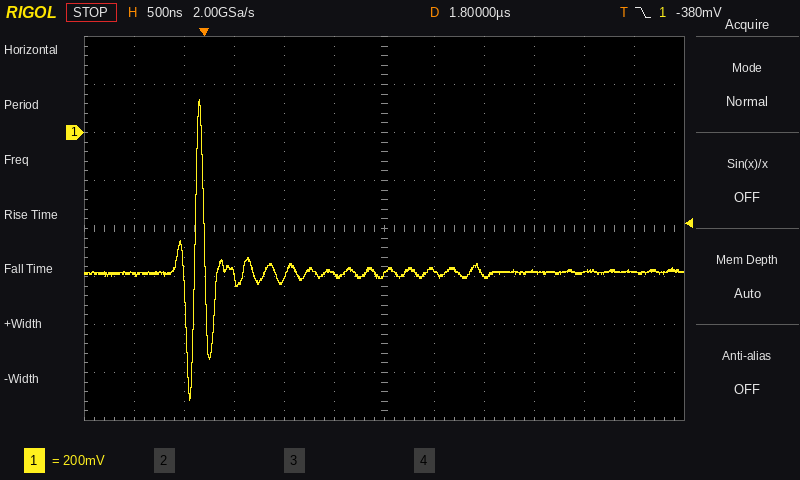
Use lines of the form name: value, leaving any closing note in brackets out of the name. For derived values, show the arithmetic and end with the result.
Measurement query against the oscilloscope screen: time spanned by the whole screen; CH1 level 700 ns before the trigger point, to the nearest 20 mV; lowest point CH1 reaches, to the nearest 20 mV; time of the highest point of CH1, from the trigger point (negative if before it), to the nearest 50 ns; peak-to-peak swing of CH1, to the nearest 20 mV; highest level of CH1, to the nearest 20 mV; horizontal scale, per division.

time spanned by the whole screen: 6 µs
CH1 level 700 ns before the trigger point, to the nearest 20 mV: -600 mV
lowest point CH1 reaches, to the nearest 20 mV: -1.12 V
time of the highest point of CH1, from the trigger point (negative if before it), to the nearest 50 ns: -50 ns
peak-to-peak swing of CH1, to the nearest 20 mV: 140 mV − (-1.12 V) = 1.26 V
highest level of CH1, to the nearest 20 mV: 140 mV
horizontal scale, per division: 500 ns
